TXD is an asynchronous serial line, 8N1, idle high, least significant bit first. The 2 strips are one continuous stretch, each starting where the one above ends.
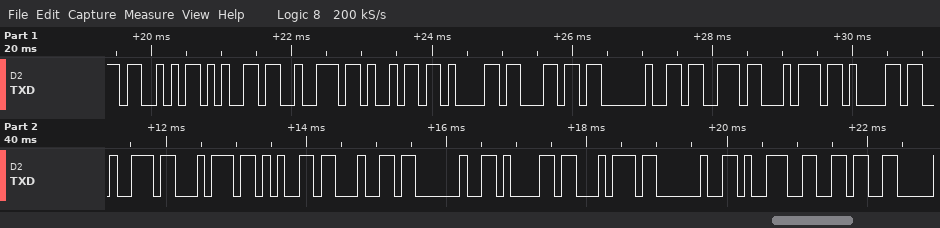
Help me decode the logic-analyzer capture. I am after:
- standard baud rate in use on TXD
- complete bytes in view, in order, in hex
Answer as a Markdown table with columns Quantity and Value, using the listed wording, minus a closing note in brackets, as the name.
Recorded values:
| Quantity | Value |
|---|---|
| standard baud rate in use on TXD | 9600 baud |
| complete bytes in view, in order, in hex | 53 65 72 69 61 6C 20 73 74 61 72 74 65 64 20 61 74 20 39 36 |
